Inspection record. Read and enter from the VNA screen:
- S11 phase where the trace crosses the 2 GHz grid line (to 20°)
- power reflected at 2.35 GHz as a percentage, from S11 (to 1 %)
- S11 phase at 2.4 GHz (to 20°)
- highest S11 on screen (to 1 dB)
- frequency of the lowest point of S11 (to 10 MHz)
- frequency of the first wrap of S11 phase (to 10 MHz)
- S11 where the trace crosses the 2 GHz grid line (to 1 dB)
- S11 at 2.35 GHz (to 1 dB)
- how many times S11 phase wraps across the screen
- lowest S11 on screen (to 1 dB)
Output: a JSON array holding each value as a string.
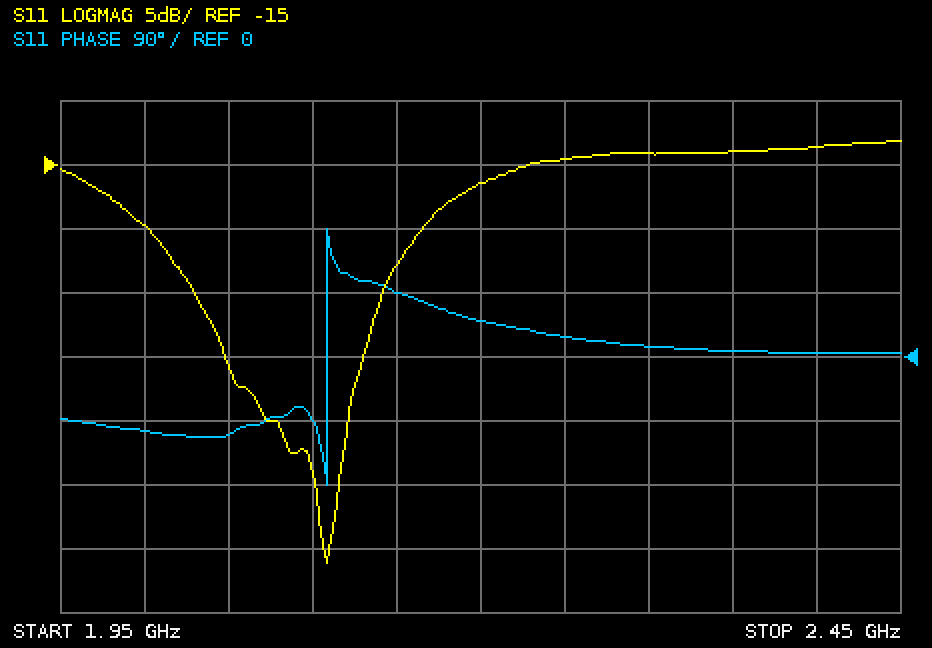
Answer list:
["-100°", "4 %", "0°", "-13 dB", "2.11 GHz", "2.11 GHz", "-20 dB", "-14 dB", "1", "-46 dB"]
